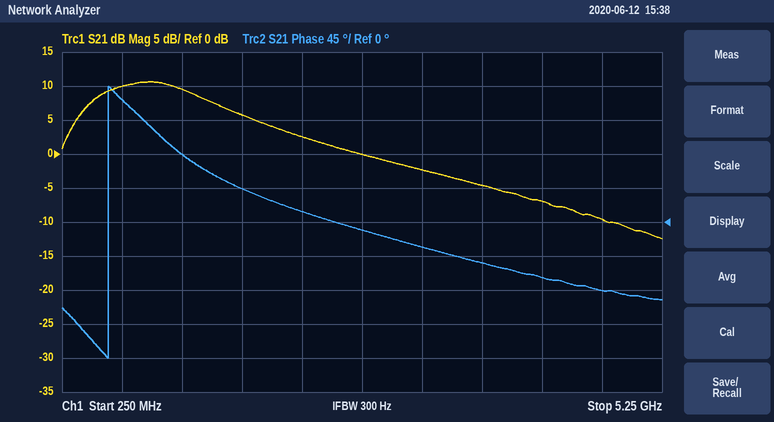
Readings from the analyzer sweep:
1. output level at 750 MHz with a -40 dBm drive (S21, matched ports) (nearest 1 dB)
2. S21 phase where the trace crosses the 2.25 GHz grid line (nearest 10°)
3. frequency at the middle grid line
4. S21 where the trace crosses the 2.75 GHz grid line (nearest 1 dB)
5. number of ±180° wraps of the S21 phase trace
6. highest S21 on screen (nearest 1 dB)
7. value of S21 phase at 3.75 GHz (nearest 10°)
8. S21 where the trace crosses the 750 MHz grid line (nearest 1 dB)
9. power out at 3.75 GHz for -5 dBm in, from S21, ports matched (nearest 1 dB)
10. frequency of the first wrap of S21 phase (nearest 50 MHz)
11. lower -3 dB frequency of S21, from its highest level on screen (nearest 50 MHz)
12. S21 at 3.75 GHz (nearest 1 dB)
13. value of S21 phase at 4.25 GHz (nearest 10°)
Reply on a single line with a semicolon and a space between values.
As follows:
-30 dBm; 10°; 2.75 GHz; 0 dB; 1; 11 dB; -50°; 10 dB; -10 dBm; 650 MHz; 500 MHz; -5 dB; -70°
